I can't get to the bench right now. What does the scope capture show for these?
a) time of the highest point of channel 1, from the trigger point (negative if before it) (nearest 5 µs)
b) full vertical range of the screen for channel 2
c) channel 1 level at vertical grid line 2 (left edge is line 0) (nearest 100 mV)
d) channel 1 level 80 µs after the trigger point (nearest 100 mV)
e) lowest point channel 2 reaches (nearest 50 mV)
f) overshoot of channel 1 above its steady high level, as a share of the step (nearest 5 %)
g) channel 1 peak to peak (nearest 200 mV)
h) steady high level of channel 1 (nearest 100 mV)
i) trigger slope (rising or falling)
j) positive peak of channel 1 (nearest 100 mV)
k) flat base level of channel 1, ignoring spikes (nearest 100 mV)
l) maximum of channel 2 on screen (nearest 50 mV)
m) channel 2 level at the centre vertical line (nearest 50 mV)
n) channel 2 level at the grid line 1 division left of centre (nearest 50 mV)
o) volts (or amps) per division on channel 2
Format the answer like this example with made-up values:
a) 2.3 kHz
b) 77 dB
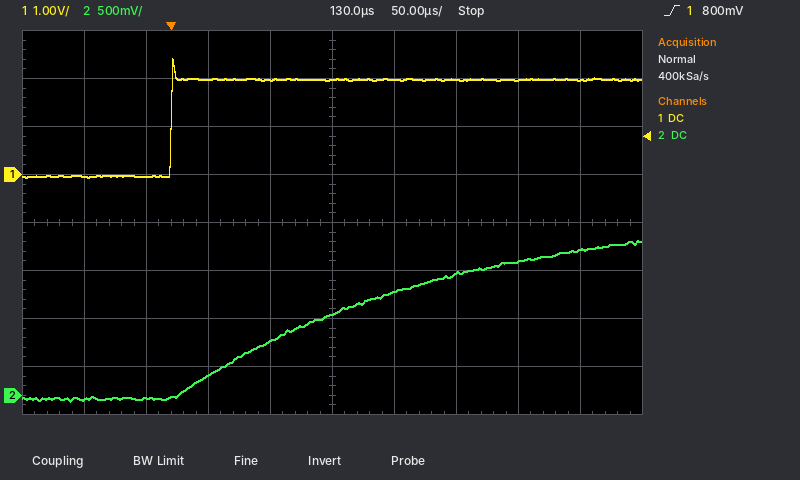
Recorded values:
a) 0 µs
b) 4 V
c) 0.0 V
d) 2.0 V
e) -50 mV
f) 20 %
g) 2.4 V
h) 2.0 V
i) rising
j) 2.4 V
k) 0.0 V
l) 1.60 V
m) 850 mV
n) 550 mV
o) 500 mV
